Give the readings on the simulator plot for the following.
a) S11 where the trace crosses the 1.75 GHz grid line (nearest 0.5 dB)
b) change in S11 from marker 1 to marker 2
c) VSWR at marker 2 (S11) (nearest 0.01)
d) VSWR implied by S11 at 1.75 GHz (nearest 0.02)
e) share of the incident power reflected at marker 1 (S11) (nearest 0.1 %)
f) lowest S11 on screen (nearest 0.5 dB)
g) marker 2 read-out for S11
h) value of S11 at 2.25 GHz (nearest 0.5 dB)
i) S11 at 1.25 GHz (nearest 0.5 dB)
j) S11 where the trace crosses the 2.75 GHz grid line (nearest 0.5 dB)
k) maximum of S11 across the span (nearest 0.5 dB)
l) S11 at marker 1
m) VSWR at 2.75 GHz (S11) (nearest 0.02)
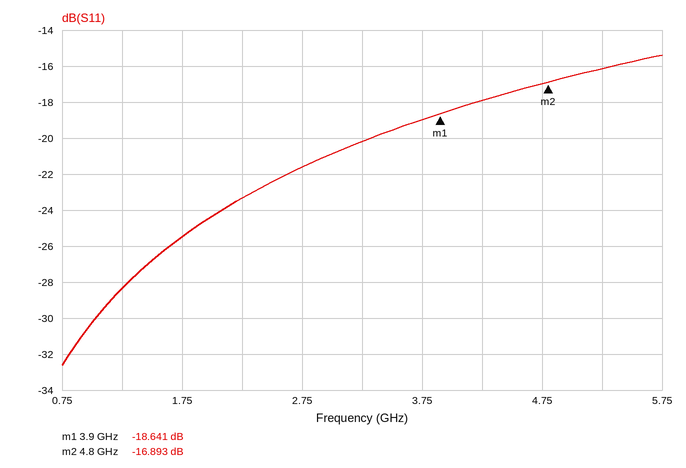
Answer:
-25.5 dB
1.748 dB
1.33
1.12
1.4 %
-32.5 dB
-16.893 dB
-23.5 dB
-28.5 dB
-21.5 dB
-15.5 dB
-18.641 dB
1.18
